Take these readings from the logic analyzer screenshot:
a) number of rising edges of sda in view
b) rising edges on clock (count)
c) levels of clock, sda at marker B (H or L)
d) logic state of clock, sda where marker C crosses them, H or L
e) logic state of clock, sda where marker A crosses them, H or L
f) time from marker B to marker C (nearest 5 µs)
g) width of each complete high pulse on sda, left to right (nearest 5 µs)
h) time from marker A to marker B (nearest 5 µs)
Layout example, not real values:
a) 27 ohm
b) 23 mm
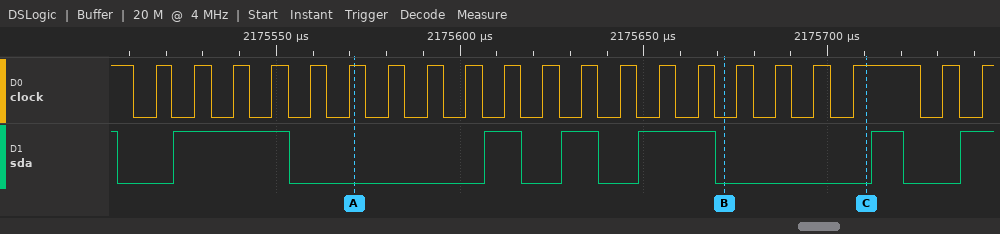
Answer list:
a) 6
b) 21
c) clock=L, sda=L
d) clock=H, sda=L
e) clock=H, sda=L
f) 40 µs
g) 30 µs, 10 µs, 10 µs, 20 µs, 10 µs
h) 100 µs
